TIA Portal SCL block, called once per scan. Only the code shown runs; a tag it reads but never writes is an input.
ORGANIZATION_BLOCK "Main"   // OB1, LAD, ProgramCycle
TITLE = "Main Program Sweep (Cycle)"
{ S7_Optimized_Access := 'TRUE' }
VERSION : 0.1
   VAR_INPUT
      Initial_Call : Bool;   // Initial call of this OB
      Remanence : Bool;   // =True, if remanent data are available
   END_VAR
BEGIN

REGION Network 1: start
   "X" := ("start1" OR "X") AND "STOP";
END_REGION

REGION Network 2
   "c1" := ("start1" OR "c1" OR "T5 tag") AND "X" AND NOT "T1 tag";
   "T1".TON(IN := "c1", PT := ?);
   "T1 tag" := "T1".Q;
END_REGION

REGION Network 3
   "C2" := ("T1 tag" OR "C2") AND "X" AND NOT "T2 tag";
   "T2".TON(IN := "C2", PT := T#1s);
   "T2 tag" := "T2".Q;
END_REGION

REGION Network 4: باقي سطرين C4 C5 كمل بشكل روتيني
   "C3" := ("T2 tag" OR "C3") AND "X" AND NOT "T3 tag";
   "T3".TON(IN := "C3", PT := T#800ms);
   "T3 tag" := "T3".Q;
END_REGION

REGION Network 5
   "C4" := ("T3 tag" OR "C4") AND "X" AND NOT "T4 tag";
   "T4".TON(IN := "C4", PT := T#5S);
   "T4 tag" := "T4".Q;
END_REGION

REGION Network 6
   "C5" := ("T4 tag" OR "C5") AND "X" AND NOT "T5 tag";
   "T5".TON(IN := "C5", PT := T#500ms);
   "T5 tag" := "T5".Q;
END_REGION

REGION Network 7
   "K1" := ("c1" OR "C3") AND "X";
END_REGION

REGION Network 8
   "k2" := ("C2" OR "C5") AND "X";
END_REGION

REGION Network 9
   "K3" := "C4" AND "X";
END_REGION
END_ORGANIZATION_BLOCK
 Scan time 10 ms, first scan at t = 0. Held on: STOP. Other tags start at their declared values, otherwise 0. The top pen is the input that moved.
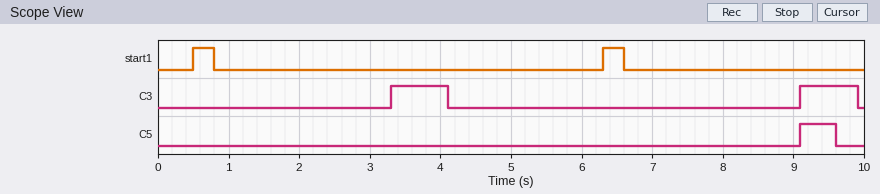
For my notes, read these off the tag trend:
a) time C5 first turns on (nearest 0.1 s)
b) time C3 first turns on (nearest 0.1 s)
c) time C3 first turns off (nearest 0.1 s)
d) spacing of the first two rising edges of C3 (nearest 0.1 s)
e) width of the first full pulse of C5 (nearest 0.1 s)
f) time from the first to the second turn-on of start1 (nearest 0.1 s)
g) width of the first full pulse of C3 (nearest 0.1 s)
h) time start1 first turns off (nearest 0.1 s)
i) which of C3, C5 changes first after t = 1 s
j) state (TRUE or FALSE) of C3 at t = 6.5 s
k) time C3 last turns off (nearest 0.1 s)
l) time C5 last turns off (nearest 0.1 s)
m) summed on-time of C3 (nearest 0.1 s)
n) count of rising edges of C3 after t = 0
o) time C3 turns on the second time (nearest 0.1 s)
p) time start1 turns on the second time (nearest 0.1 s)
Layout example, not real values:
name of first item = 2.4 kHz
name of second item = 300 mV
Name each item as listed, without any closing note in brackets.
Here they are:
time C5 first turns on = 9.1 s
time C3 first turns on = 3.3 s
time C3 first turns off = 4.1 s
spacing of the first two rising edges of C3 = 5.8 s
width of the first full pulse of C5 = 0.5 s
time from the first to the second turn-on of start1 = 5.8 s
width of the first full pulse of C3 = 0.8 s
time start1 first turns off = 0.8 s
which of C3, C5 changes first after t = 1 s = C3
state (TRUE or FALSE) of C3 at t = 6.5 s = FALSE
time C3 last turns off = 9.9 s
time C5 last turns off = 9.6 s
summed on-time of C3 = 1.6 s
count of rising edges of C3 after t = 0 = 2
time C3 turns on the second time = 9.1 s
time start1 turns on the second time = 6.3 s
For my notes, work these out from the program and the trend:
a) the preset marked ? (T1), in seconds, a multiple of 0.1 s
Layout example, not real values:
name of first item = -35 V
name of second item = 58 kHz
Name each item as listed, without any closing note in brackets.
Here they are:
the preset marked ? (T1), in seconds, a multiple of 0.1 s = 1.8 s
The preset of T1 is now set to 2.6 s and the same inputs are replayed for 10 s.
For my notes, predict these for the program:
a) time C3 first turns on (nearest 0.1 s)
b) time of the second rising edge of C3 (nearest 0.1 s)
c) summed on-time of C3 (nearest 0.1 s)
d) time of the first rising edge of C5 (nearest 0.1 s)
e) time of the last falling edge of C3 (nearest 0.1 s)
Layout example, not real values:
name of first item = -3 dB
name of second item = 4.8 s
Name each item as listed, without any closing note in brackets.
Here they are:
time C3 first turns on = 4.1 s
time of the second rising edge of C3 = 9.9 s
summed on-time of C3 = 0.9 s
time of the first rising edge of C5 = 9.9 s
time of the last falling edge of C3 = 4.9 s
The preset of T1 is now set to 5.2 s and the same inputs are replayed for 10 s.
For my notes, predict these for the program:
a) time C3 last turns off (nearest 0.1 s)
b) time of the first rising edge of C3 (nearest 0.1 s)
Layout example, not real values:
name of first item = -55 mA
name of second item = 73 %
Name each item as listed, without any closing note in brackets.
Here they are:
time C3 last turns off = 7.5 s
time of the first rising edge of C3 = 6.7 s
